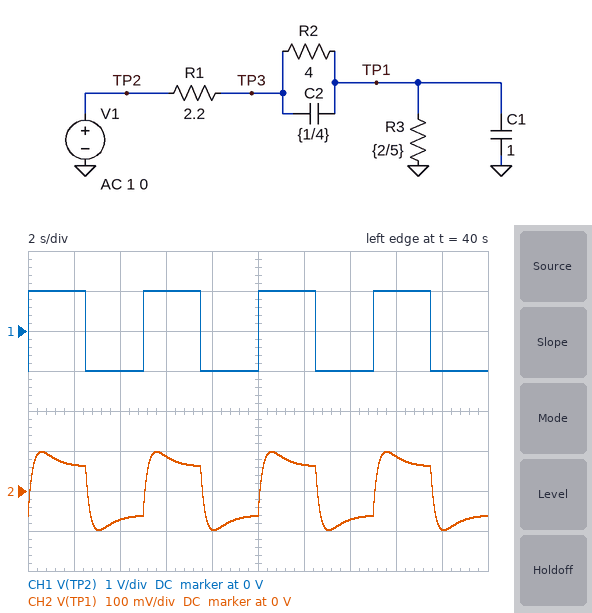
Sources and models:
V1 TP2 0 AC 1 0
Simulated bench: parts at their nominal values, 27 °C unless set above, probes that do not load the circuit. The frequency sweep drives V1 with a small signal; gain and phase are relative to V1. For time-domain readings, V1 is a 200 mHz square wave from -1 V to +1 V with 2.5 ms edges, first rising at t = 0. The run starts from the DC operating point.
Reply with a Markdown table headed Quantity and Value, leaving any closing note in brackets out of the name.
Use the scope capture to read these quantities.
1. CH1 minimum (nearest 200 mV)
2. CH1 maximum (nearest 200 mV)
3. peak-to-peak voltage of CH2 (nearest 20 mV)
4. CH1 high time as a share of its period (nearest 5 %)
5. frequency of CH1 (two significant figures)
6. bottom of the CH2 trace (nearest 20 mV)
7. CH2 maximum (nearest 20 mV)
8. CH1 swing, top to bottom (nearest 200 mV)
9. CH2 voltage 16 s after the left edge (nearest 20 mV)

| Quantity | Value |
|---|---|
| CH1 minimum | -1.0 V |
| CH1 maximum | 1.0 V |
| peak-to-peak voltage of CH2 | 200 mV |
| CH1 high time as a share of its period | 50 % |
| frequency of CH1 | 200 mHz |
| bottom of the CH2 trace | -100 mV |
| CH2 maximum | 100 mV |
| CH1 swing, top to bottom | 2.0 V |
| CH2 voltage 16 s after the left edge | 80 mV |
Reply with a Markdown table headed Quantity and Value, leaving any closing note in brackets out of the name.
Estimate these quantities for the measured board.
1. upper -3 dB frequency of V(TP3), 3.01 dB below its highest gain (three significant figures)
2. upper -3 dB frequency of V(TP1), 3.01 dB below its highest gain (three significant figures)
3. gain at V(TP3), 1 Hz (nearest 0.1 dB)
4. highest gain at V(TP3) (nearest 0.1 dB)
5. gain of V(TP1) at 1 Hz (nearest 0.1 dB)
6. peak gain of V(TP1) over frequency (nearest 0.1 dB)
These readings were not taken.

| Quantity | Value |
|---|---|
| upper -3 dB frequency of V(TP3), 3.01 dB below its highest gain | 512 mHz |
| upper -3 dB frequency of V(TP1), 3.01 dB below its highest gain | 998 mHz |
| gain at V(TP3), 1 Hz | -10.1 dB |
| highest gain at V(TP3) | -3.5 dB |
| gain of V(TP1) at 1 Hz | -24.5 dB |
| peak gain of V(TP1) over frequency | -21.4 dB |
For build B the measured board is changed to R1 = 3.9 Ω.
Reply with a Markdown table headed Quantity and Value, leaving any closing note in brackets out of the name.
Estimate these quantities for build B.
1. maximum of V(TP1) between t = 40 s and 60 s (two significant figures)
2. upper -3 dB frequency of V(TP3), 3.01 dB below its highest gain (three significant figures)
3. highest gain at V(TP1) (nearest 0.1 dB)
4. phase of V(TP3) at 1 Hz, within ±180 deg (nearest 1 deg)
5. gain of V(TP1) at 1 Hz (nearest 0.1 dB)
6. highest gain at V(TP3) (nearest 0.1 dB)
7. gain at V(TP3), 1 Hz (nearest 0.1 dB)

| Quantity | Value |
|---|---|
| maximum of V(TP1) between t = 40 s and 60 s | 66 mV |
| upper -3 dB frequency of V(TP3), 3.01 dB below its highest gain | 358 mHz |
| highest gain at V(TP1) | -24.5 dB |
| phase of V(TP3) at 1 Hz, within ±180 deg | -68 deg |
| gain of V(TP1) at 1 Hz | -28.9 dB |
| highest gain at V(TP3) | -5.5 dB |
| gain at V(TP3), 1 Hz | -14.5 dB |
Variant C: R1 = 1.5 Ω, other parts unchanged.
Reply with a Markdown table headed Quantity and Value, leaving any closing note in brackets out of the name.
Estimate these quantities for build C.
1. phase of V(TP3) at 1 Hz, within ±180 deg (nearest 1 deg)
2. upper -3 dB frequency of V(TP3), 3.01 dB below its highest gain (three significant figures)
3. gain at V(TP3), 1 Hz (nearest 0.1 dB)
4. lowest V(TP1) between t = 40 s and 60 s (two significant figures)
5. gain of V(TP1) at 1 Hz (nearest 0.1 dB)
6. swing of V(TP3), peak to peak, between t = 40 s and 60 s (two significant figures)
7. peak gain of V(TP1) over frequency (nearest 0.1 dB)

| Quantity | Value |
|---|---|
| phase of V(TP3) at 1 Hz, within ±180 deg | -54 deg |
| upper -3 dB frequency of V(TP3), 3.01 dB below its highest gain | 680 mHz |
| gain at V(TP3), 1 Hz | -7.4 dB |
| lowest V(TP1) between t = 40 s and 60 s | -120 mV |
| gain of V(TP1) at 1 Hz | -21.8 dB |
| swing of V(TP3), peak to peak, between t = 40 s and 60 s | 1.5 V |
| peak gain of V(TP1) over frequency | -19.7 dB |
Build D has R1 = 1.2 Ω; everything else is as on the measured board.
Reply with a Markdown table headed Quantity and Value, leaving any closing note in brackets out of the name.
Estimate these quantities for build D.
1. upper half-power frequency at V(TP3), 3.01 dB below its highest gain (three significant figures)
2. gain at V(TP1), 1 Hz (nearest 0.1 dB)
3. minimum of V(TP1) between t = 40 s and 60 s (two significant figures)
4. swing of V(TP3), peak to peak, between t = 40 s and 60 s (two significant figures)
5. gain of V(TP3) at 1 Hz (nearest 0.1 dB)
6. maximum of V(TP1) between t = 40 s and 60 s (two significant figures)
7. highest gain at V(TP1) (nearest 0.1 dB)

| Quantity | Value |
|---|---|
| upper half-power frequency at V(TP3), 3.01 dB below its highest gain | 812 mHz |
| gain at V(TP1), 1 Hz | -20.4 dB |
| minimum of V(TP1) between t = 40 s and 60 s | -140 mV |
| swing of V(TP3), peak to peak, between t = 40 s and 60 s | 1.6 V |
| gain of V(TP3) at 1 Hz | -6.0 dB |
| maximum of V(TP1) between t = 40 s and 60 s | 140 mV |
| highest gain at V(TP1) | -18.9 dB |
